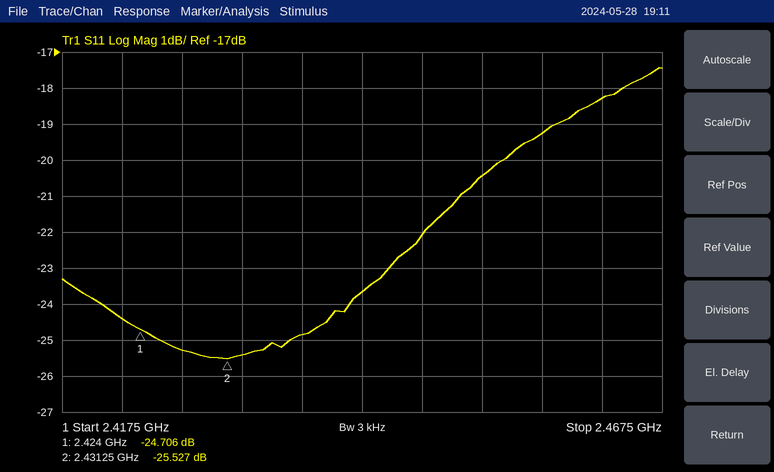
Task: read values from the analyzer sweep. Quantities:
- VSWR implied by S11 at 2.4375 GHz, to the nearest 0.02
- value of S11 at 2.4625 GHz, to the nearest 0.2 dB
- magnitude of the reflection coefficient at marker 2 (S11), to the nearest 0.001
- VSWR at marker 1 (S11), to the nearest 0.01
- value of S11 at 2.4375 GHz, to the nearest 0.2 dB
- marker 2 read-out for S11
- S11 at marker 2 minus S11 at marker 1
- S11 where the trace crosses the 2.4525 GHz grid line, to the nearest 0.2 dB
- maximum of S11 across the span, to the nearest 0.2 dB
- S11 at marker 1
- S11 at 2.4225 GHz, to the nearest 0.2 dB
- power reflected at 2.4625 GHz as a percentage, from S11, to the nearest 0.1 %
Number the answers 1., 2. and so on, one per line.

1. 1.12
2. -18.2 dB
3. 0.053
4. 1.12
5. -24.8 dB
6. -25.527 dB
7. -0.821 dB
8. -20.4 dB
9. -17.4 dB
10. -24.706 dB
11. -24.4 dB
12. 1.5 %
